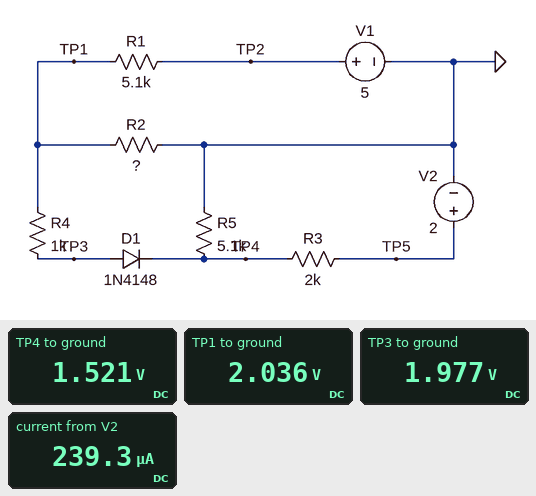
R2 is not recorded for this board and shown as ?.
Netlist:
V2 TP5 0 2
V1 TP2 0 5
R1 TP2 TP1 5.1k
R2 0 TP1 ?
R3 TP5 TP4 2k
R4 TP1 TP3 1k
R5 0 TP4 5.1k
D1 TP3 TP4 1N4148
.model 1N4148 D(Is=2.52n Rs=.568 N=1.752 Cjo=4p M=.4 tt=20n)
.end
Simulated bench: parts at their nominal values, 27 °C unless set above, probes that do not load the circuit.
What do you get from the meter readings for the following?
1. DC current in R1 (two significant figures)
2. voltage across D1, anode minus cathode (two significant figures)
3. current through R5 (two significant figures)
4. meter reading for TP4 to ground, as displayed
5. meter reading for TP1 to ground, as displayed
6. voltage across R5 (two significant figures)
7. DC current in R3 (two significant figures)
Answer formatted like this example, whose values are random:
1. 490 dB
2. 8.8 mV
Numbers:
1. 580 µA
2. 460 mV
3. 300 µA
4. 1.521 V
5. 2.036 V
6. 1.5 V
7. 240 µA
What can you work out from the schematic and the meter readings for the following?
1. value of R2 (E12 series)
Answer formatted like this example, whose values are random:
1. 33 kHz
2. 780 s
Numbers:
1. 3.9 kΩ
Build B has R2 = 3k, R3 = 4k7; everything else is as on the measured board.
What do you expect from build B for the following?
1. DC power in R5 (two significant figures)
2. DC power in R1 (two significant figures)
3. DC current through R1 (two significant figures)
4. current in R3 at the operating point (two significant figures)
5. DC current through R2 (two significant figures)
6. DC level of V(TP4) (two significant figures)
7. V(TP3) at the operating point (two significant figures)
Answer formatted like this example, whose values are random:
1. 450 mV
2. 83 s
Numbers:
1. 280 µW
2. 2.1 mW
3. 640 µA
4. 170 µA
5. 580 µA
6. 1.2 V
7. 1.7 V
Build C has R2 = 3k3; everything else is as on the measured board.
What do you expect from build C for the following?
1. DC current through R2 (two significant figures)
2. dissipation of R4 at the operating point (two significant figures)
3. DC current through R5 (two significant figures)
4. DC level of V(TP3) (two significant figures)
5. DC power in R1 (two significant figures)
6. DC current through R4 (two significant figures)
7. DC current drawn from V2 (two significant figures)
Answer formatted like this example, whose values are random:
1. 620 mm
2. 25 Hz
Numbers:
1. 580 µA
2. 620 nW
3. 290 µA
4. 1.9 V
5. 1.9 mW
6. 25 µA
7. 260 µA
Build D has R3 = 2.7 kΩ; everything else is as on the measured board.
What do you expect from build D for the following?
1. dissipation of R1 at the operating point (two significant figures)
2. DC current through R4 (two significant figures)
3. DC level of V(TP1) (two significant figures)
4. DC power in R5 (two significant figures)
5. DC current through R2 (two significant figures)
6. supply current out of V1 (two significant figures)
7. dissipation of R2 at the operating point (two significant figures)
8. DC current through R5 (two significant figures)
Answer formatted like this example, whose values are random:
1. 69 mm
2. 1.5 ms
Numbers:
1. 1.8 mW
2. 78 µA
3. 2.0 V
4. 410 µW
5. 510 µA
6. 590 µA
7. 1.0 mW
8. 280 µA
